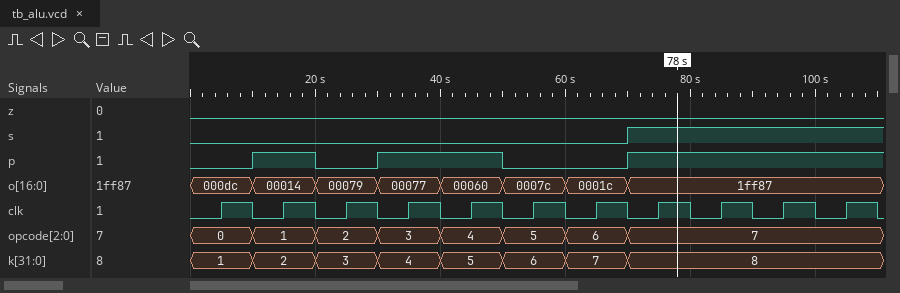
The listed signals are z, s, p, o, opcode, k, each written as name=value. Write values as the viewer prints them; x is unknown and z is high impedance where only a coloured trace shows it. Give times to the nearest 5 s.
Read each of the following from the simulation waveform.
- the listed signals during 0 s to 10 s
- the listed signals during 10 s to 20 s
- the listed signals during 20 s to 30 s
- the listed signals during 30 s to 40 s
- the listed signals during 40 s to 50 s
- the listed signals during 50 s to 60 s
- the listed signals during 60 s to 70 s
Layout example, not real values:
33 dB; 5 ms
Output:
z=0, s=0, p=0, o=000dc, opcode=0, k=1; z=0, s=0, p=1, o=00014, opcode=1, k=2; z=0, s=0, p=0, o=00079, opcode=2, k=3; z=0, s=0, p=1, o=00077, opcode=3, k=4; z=0, s=0, p=1, o=00060, opcode=4, k=5; z=0, s=0, p=0, o=0007c, opcode=5, k=6; z=0, s=0, p=0, o=0001c, opcode=6, k=7
